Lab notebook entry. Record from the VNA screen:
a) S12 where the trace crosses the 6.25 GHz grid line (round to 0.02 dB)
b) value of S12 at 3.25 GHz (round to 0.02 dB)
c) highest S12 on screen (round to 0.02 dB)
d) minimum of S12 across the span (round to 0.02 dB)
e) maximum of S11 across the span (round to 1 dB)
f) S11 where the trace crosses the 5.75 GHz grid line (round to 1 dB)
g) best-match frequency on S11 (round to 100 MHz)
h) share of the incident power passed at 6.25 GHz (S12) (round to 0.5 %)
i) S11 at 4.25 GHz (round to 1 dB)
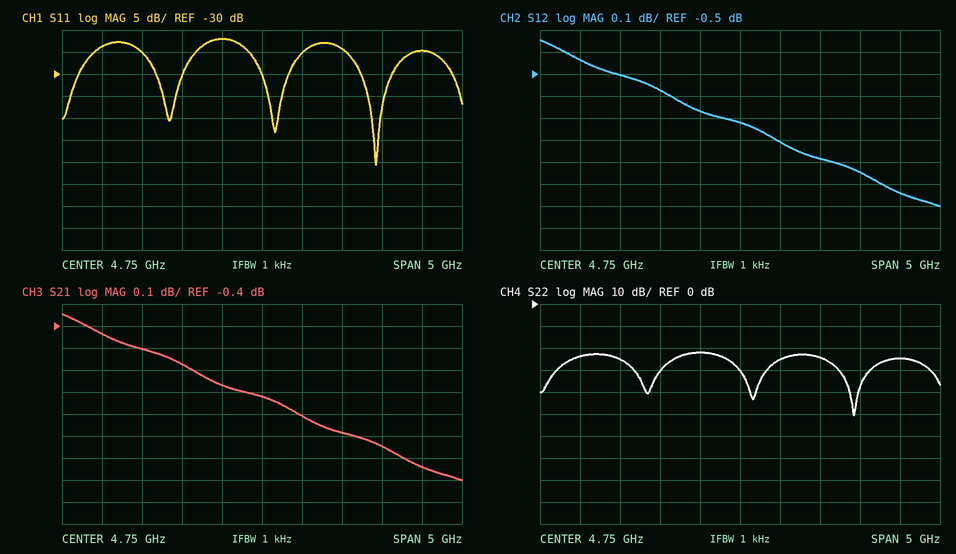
-0.94 dB
-0.50 dB
-0.34 dB
-1.10 dB
-22 dB
-24 dB
6.2 GHz
80.5 %
-22 dB
